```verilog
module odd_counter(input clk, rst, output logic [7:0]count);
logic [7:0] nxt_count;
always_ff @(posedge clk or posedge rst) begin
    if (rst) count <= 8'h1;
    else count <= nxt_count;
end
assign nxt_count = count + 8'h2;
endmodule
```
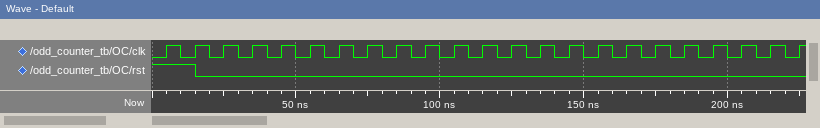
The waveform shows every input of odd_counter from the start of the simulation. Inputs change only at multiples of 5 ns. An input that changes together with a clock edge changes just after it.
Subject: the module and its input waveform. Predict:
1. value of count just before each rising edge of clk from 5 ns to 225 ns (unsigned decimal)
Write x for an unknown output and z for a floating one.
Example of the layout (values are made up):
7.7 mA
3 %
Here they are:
1, 1, 1, 3, 5, 7, 9, 11, 13, 15, 17, 19, 21, 23, 25, 27, 29, 31, 33, 35, 37, 39, 41
